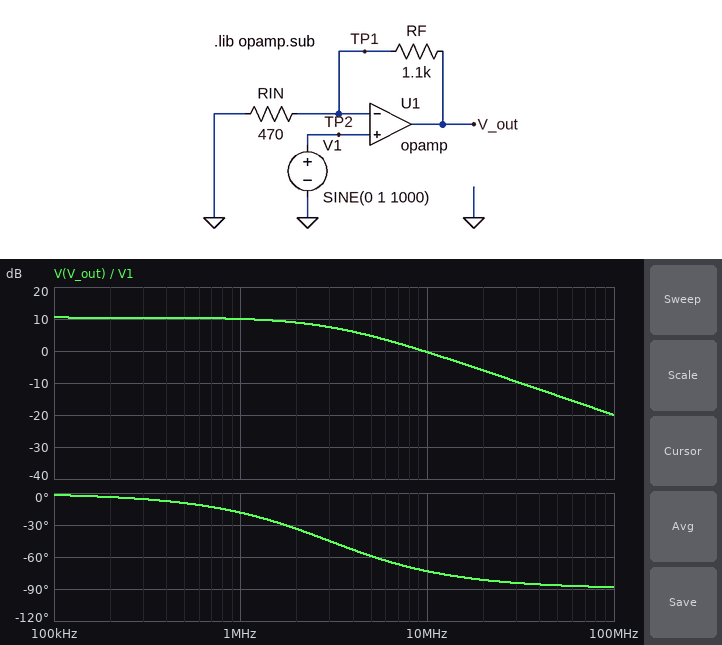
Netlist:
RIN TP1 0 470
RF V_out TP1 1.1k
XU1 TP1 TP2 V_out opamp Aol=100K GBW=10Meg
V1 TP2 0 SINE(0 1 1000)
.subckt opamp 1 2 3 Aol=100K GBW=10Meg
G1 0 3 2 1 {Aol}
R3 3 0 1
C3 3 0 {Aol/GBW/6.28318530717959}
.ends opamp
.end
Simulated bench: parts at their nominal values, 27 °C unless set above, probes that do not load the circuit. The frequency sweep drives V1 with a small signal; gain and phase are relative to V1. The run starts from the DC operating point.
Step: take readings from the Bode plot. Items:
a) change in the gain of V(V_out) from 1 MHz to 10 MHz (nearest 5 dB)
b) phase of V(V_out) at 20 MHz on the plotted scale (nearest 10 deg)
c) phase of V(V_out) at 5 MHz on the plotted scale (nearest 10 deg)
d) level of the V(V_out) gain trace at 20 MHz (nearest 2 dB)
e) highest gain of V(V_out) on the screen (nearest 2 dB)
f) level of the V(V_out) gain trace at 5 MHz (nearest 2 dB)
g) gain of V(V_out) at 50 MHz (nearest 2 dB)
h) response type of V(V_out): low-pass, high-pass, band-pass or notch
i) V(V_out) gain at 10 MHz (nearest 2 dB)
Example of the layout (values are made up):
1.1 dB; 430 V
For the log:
-10 dB; -80 deg; -60 deg; -6 dB; 10 dB; 4 dB; -14 dB; low-pass; 0 dB
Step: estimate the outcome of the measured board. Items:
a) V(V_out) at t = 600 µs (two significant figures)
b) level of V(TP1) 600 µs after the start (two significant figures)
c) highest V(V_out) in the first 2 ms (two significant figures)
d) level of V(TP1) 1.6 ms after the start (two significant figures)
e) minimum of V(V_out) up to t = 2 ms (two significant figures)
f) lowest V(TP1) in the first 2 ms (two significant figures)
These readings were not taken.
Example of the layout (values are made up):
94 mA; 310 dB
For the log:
-2.0 V; -590 mV; 3.3 V; -590 mV; -3.3 V; -1.0 V
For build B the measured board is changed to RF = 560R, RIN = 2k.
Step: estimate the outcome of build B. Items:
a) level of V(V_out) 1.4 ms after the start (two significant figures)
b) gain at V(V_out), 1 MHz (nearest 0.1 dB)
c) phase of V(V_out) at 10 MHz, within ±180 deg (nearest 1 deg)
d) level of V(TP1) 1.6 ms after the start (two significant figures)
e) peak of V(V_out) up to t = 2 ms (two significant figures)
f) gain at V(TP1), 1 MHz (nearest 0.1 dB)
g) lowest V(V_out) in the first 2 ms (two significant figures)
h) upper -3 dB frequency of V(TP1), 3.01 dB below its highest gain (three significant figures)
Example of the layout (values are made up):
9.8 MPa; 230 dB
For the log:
750 mV; 2.1 dB; -52 deg; -590 mV; 1.3 V; -0.1 dB; -1.3 V; 7.81 MHz
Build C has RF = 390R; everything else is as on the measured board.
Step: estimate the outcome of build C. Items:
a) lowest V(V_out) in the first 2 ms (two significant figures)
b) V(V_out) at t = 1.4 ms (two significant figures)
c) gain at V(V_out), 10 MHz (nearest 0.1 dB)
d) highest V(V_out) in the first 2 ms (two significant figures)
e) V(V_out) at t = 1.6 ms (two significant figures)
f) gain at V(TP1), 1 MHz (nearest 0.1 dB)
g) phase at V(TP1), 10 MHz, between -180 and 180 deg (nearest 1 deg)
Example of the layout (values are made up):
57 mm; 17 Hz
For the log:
-1.8 V; 1.1 V; -1.1 dB; 1.8 V; -1.1 V; -0.1 dB; -61 deg
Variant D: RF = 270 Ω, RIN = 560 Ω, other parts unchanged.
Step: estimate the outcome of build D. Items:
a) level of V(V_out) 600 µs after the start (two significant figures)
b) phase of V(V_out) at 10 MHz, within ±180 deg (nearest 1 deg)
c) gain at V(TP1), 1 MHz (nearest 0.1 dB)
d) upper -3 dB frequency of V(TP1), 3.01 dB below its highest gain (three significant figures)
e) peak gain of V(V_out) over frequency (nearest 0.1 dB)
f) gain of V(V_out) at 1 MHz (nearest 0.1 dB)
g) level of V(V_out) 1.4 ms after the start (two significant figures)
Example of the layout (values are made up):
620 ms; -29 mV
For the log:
-870 mV; -56 deg; -0.1 dB; 6.75 MHz; 3.4 dB; 3.3 dB; 870 mV
